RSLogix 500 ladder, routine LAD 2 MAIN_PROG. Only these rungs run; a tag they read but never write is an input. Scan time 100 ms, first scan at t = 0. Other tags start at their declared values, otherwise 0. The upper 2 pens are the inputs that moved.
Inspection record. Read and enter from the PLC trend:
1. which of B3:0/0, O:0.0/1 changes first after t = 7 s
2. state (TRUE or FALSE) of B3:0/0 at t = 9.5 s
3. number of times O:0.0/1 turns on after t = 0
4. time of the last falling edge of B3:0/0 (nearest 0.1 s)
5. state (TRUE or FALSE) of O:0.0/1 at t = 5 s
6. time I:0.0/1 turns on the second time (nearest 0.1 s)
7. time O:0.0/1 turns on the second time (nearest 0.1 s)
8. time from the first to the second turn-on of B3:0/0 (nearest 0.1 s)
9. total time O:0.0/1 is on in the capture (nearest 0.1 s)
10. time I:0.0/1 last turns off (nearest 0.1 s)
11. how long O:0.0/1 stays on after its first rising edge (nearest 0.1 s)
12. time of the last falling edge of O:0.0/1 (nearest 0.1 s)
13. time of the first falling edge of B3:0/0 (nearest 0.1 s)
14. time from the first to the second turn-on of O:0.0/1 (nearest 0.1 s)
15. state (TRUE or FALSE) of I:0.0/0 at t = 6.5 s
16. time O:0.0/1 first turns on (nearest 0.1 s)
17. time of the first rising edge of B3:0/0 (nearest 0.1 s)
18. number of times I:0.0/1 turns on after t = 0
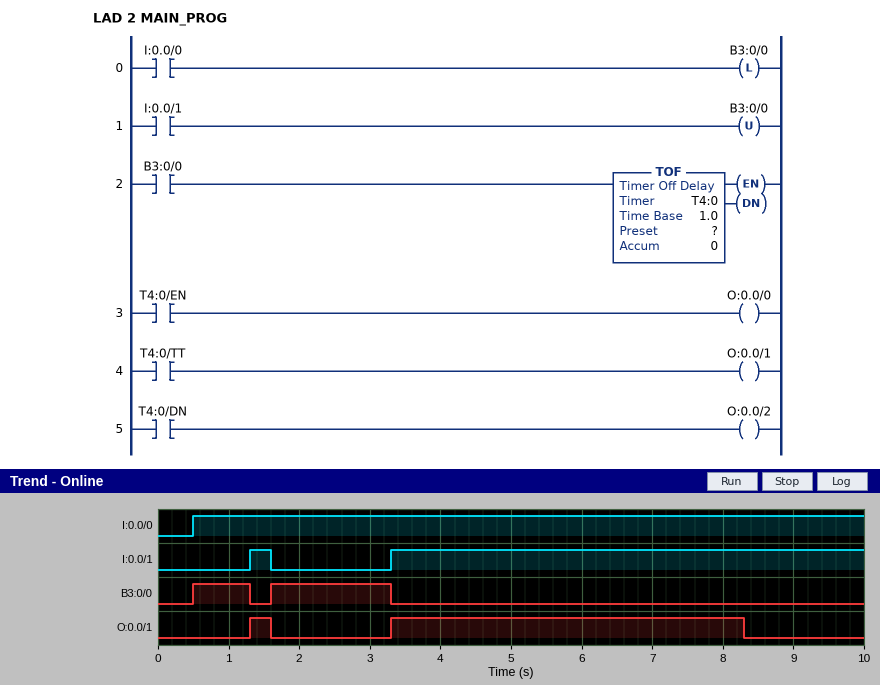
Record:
O:0.0/1
FALSE
2
3.3 s
TRUE
3.3 s
3.3 s
1.1 s
5.3 s
1.6 s
0.3 s
8.3 s
1.3 s
2.0 s
TRUE
1.3 s
0.5 s
2
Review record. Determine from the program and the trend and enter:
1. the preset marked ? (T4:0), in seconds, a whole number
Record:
5 s
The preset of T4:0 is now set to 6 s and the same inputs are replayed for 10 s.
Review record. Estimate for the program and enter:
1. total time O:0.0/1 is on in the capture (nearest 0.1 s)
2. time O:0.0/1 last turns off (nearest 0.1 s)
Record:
6.3 s
9.3 s
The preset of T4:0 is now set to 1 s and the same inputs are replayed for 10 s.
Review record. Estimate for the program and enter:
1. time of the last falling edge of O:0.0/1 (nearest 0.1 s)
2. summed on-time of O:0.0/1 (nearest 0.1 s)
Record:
4.3 s
1.3 s
